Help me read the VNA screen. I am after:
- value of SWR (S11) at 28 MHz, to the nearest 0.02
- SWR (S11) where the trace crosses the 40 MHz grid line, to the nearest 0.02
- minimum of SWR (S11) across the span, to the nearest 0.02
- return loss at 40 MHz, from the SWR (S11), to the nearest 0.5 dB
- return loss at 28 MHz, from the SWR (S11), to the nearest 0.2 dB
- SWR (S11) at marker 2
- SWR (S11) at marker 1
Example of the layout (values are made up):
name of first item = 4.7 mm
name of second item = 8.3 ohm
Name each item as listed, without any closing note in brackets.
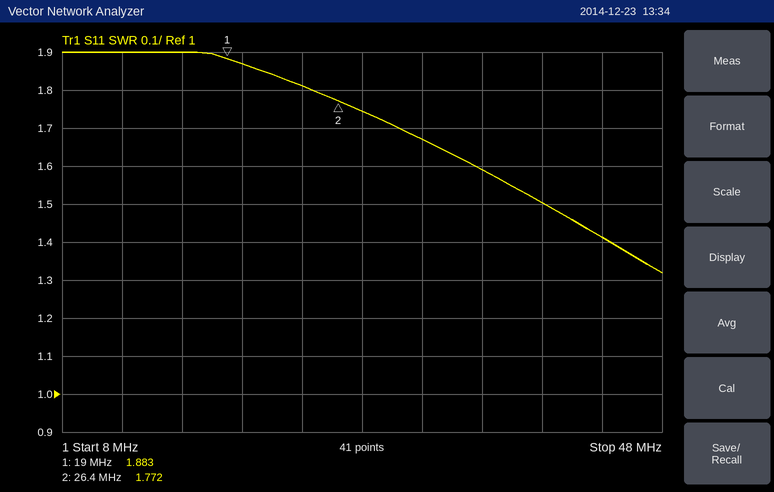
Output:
value of SWR (S11) at 28 MHz, to the nearest 0.02 = 1.74
SWR (S11) where the trace crosses the 40 MHz grid line, to the nearest 0.02 = 1.50
minimum of SWR (S11) across the span, to the nearest 0.02 = 1.32
return loss at 40 MHz, from the SWR (S11), to the nearest 0.5 dB = 14.0 dB
return loss at 28 MHz, from the SWR (S11), to the nearest 0.2 dB = 11.4 dB
SWR (S11) at marker 2 = 1.772
SWR (S11) at marker 1 = 1.883
